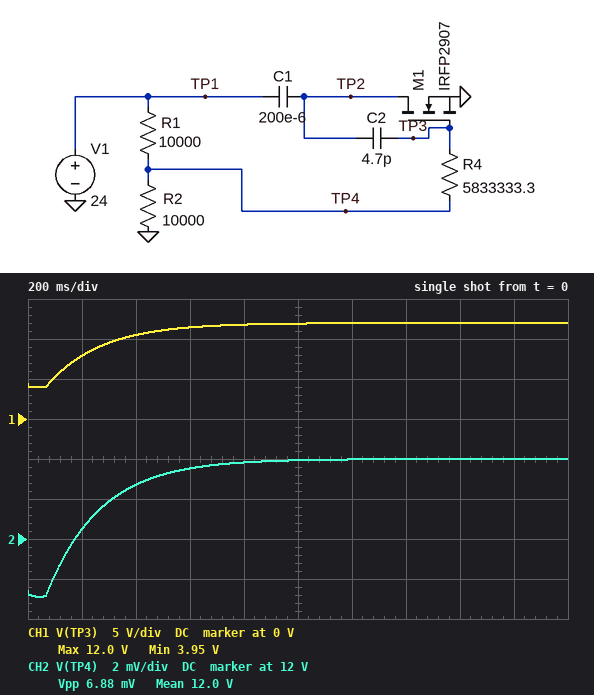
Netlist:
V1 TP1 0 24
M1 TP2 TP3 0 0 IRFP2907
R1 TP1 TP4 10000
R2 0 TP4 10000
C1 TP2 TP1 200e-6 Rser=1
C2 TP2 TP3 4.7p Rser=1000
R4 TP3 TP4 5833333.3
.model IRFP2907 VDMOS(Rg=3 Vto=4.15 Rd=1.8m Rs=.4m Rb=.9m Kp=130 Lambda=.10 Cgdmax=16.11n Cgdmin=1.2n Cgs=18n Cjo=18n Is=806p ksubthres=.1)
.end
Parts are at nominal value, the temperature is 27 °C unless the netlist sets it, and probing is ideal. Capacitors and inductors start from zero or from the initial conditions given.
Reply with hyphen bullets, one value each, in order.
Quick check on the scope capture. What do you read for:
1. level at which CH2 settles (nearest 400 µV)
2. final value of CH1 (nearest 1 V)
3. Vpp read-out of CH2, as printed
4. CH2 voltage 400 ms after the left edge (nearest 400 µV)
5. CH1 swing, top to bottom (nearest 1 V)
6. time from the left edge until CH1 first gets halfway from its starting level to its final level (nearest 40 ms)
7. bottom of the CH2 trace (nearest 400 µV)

- 12.0000 V
- 12 V
- 6.88 mV
- 11.9988 V
- 8 V
- 200 ms
- 11.9932 V
